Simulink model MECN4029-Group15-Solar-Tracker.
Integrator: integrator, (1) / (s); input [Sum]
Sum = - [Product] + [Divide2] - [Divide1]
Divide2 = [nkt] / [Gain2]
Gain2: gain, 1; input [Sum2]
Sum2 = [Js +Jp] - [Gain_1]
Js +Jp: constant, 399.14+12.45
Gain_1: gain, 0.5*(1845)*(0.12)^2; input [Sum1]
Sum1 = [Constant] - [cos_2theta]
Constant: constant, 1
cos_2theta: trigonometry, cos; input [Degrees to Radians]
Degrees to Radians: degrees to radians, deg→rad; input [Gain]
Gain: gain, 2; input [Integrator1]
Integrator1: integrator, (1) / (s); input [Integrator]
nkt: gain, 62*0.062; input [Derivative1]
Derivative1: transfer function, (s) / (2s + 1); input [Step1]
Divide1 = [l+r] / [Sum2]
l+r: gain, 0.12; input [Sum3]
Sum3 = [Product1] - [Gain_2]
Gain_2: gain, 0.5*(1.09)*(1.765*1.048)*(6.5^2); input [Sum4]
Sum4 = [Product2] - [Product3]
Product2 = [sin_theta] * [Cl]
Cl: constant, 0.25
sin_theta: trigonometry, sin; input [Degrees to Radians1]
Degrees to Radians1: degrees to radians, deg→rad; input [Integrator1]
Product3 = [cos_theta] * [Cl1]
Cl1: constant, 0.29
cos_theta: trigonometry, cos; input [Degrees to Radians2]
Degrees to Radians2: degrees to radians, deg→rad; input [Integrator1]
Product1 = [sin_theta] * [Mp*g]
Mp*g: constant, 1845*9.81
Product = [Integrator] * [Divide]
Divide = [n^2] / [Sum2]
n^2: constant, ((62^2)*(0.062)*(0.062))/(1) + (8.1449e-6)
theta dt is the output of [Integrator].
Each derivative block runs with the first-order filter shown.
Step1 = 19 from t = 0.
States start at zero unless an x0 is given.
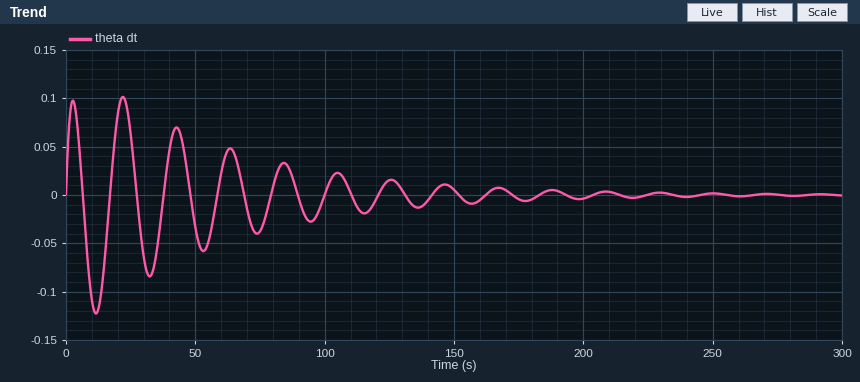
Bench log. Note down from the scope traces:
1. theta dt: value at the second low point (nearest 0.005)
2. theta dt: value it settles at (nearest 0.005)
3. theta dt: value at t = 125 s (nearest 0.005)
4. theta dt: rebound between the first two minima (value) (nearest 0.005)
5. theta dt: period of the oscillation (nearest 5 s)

-0.085
0.000
0.015
0.100
20 s
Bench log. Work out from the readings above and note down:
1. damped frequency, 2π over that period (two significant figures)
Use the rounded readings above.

0.31 rad/s
